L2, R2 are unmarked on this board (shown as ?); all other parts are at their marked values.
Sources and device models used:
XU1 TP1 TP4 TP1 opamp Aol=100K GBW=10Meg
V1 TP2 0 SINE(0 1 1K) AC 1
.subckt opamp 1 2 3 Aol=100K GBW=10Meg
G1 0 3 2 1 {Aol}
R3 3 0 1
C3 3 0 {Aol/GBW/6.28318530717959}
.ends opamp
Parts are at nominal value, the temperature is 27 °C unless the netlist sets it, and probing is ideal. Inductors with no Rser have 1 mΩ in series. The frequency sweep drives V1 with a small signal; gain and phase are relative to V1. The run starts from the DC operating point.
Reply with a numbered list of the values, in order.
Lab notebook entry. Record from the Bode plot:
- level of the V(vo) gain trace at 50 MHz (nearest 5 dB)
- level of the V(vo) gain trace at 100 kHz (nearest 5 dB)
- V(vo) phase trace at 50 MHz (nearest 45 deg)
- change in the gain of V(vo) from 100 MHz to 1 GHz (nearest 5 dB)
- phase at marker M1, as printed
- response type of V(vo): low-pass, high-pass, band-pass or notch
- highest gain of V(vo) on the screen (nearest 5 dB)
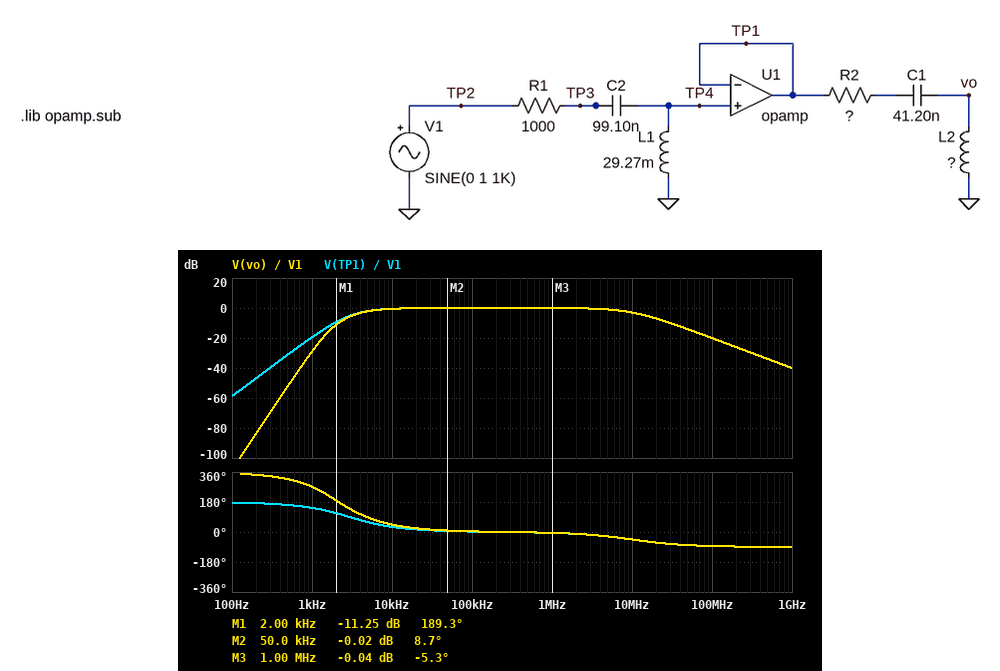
1. -15 dB
2. 0 dB
3. -90 deg
4. -20 dB
5. 189.3 deg
6. band-pass
7. 0 dB
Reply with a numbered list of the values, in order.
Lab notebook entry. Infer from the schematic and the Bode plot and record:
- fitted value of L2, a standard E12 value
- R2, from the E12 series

1. 220 mH
2. 3.3 kΩ
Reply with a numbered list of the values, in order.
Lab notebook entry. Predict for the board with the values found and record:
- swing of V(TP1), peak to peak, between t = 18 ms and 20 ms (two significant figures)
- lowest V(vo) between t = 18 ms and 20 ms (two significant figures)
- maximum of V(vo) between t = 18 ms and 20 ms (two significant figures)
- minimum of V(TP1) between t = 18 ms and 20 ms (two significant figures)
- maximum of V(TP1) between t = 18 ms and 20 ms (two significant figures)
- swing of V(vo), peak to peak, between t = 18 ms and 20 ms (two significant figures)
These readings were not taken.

1. 210 mV
2. -35 mV
3. 35 mV
4. -110 mV
5. 110 mV
6. 71 mV
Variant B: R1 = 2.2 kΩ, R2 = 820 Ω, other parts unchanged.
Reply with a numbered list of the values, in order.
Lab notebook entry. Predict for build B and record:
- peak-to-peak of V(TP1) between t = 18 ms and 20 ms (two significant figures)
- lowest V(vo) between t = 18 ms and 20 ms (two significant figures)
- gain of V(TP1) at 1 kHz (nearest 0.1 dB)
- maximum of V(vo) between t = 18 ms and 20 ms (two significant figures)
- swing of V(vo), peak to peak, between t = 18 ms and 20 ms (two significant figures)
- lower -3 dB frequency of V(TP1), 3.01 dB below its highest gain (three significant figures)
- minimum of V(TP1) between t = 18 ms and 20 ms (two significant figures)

1. 140 mV
2. -37 mV
3. -23.1 dB
4. 37 mV
5. 74 mV
6. 11.2 kHz
7. -70 mV
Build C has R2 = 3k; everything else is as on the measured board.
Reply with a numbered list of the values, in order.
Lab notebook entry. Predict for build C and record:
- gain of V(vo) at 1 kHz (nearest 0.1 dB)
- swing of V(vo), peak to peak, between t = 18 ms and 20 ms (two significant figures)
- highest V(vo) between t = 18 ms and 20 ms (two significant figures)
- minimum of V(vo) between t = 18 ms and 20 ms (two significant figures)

1. -28.5 dB
2. 75 mV
3. 38 mV
4. -38 mV
